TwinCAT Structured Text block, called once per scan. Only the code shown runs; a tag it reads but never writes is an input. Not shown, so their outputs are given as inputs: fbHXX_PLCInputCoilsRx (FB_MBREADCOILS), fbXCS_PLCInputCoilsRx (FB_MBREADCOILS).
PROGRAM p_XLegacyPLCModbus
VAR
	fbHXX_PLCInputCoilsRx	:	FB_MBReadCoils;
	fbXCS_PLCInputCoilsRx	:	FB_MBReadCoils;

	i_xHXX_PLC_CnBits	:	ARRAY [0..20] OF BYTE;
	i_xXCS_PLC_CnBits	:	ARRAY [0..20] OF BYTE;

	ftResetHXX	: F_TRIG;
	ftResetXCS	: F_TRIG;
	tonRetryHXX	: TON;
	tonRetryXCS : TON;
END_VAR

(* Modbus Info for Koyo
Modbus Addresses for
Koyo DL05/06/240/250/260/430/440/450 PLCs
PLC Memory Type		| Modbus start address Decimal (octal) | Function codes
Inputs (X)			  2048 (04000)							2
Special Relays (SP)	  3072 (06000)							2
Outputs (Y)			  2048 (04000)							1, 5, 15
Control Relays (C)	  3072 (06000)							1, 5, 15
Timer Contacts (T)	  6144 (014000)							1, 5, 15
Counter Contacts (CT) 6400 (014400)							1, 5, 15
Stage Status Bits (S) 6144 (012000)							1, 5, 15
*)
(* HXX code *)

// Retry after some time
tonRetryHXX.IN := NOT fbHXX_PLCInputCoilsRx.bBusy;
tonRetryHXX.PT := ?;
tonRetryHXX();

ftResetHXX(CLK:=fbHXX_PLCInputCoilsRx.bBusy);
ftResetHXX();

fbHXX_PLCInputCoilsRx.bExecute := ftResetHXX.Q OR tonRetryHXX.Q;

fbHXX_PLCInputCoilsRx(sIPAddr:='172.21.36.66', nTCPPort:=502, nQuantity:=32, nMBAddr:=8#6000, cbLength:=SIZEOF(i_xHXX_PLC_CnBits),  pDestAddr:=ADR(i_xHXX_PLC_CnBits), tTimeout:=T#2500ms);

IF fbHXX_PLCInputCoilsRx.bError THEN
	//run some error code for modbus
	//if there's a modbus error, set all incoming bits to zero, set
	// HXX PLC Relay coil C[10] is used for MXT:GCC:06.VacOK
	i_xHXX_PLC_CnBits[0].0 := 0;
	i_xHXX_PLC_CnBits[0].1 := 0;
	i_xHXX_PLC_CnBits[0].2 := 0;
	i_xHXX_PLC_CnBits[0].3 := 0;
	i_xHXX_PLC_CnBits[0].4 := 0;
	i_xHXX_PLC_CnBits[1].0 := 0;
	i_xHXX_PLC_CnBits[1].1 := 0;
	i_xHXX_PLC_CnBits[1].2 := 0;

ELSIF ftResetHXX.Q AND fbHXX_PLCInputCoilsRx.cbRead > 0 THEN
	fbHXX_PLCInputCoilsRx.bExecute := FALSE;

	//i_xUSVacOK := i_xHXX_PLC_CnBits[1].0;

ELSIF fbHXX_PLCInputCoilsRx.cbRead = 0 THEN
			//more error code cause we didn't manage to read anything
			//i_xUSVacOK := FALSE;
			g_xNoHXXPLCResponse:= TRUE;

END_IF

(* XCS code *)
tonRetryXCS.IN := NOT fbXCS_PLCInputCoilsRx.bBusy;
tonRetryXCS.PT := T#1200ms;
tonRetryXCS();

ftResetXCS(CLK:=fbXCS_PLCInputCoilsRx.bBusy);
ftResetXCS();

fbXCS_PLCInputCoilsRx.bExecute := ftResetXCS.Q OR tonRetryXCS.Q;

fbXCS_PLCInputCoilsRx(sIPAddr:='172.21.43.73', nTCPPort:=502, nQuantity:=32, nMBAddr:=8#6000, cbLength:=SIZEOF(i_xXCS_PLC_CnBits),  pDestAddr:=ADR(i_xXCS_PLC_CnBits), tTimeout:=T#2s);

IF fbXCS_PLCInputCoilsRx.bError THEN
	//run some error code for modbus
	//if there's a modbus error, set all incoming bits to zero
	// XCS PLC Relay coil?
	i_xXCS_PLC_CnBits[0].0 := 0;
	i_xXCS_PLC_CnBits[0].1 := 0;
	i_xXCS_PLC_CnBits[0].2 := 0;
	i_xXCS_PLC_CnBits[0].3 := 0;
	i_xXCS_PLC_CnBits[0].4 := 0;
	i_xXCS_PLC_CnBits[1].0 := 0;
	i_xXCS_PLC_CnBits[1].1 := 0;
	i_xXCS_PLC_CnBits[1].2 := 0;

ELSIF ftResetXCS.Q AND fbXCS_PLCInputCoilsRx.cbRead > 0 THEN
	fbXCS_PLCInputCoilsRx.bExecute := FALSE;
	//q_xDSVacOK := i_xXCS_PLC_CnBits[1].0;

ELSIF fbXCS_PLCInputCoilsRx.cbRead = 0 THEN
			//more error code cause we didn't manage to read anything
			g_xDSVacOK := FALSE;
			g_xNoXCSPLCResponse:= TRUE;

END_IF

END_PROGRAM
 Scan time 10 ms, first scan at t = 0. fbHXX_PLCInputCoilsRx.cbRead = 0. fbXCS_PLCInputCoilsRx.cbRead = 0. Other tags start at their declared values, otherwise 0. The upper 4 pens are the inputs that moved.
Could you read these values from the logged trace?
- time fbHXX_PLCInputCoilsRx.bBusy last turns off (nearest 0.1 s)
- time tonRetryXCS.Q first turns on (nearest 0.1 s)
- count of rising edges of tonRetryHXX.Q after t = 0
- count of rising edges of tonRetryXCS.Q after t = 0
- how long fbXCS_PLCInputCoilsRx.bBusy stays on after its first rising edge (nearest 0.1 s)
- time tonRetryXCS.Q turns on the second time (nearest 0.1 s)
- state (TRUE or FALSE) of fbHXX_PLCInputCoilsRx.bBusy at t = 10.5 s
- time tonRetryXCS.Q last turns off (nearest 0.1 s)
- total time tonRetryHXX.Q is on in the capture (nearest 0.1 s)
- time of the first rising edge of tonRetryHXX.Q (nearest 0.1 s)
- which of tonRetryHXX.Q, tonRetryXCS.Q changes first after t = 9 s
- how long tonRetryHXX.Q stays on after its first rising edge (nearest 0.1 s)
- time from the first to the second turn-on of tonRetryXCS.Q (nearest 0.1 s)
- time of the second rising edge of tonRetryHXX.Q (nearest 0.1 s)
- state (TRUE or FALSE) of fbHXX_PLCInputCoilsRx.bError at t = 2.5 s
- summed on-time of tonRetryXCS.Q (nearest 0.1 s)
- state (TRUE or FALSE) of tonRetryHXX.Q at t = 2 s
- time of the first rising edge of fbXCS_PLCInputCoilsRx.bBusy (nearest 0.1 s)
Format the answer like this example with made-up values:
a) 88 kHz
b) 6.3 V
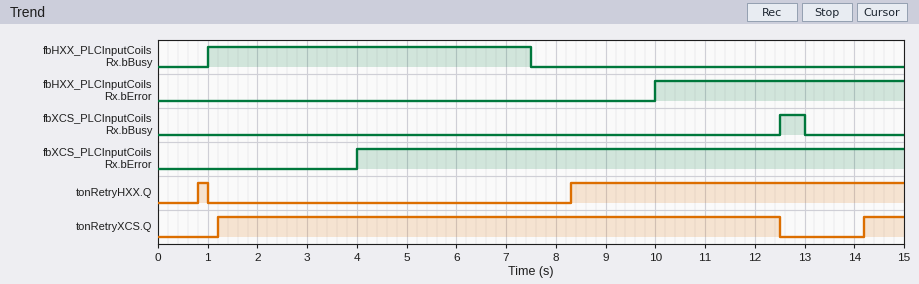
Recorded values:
a) 7.5 s
b) 1.2 s
c) 2
d) 2
e) 0.5 s
f) 14.2 s
g) FALSE
h) 12.5 s
i) 6.9 s
j) 0.8 s
k) tonRetryXCS.Q
l) 0.2 s
m) 13.0 s
n) 8.3 s
o) FALSE
p) 12.1 s
q) FALSE
r) 12.5 s
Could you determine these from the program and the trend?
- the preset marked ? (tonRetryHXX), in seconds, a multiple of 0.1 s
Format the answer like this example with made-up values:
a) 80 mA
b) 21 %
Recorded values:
a) 0.8 s
